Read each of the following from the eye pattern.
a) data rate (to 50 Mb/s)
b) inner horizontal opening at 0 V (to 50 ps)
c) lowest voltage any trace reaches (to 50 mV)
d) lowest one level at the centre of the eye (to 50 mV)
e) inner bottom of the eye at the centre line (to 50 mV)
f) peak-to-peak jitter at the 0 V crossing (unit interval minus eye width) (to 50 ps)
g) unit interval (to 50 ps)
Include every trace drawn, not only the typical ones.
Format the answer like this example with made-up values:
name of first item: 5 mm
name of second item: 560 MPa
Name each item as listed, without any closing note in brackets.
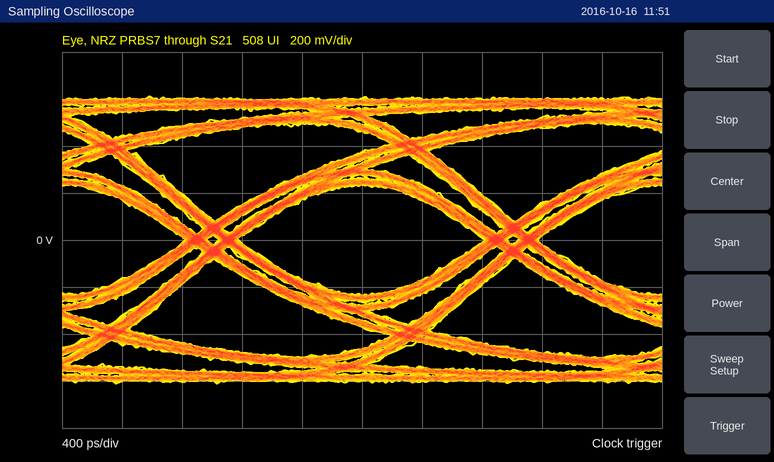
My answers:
data rate: 500 Mb/s
inner horizontal opening at 0 V: 1.65 ns
lowest voltage any trace reaches: -600 mV
lowest one level at the centre of the eye: 250 mV
inner bottom of the eye at the centre line: -250 mV
peak-to-peak jitter at the 0 V crossing (unit interval minus eye width): 350 ps
unit interval: 2.00 ns
